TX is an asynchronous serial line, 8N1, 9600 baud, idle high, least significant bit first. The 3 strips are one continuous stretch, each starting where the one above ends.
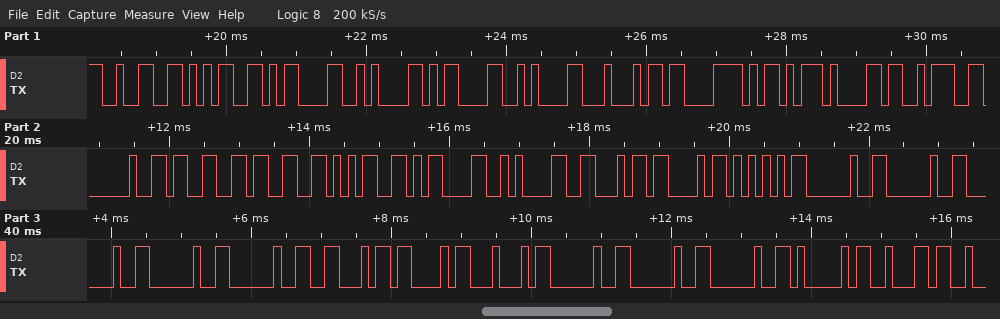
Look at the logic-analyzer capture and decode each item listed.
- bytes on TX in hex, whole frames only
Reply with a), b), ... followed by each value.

a) 32 35 0D 0A 0D 0A 44 C3 AD 61 3A 20 33 33 35 0D 0A 46 43 55 20 20 20 20 20 46 43 44 20 20 20 41 62
